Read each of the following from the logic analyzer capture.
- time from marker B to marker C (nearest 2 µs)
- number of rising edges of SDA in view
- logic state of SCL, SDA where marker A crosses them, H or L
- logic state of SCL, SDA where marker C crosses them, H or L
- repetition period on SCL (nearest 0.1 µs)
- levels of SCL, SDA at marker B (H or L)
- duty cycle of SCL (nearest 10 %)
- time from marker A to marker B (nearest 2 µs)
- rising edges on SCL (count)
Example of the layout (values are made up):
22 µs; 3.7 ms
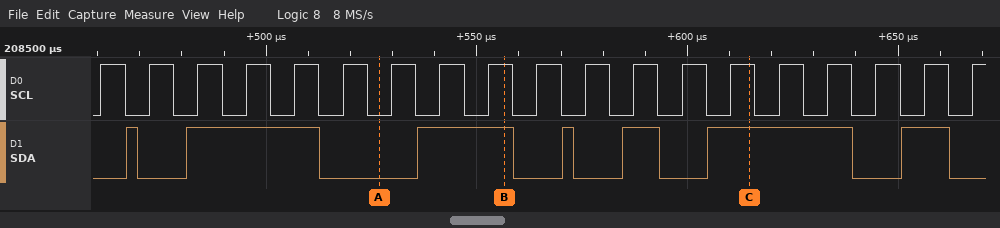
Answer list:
58 µs; 7; SCL=L, SDA=L; SCL=H, SDA=H; 11.5 µs; SCL=H, SDA=H; 50 %; 30 µs; 19
